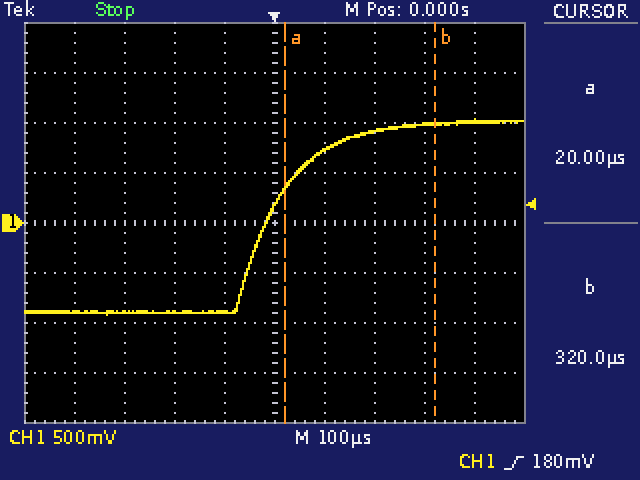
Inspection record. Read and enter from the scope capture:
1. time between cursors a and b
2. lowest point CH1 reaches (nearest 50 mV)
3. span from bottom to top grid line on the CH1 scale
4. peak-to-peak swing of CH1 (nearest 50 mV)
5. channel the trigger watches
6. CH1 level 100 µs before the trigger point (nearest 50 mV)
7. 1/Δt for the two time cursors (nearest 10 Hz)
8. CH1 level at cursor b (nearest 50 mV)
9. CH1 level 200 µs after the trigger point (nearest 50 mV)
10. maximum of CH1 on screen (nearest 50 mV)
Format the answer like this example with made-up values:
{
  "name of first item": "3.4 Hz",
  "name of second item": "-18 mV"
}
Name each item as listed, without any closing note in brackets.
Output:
{
  "time between cursors a and b": "300 µs",
  "lowest point CH1 reaches": "-900 mV",
  "span from bottom to top grid line on the CH1 scale": "4 V",
  "peak-to-peak swing of CH1": "1.95 V",
  "channel the trigger watches": "CH1",
  "CH1 level 100 µs before the trigger point": "-900 mV",
  "1/Δt for the two time cursors": "3.33 kHz",
  "CH1 level at cursor b": "1.00 V",
  "CH1 level 200 µs after the trigger point": "900 mV",
  "maximum of CH1 on screen": "1.05 V"
}
